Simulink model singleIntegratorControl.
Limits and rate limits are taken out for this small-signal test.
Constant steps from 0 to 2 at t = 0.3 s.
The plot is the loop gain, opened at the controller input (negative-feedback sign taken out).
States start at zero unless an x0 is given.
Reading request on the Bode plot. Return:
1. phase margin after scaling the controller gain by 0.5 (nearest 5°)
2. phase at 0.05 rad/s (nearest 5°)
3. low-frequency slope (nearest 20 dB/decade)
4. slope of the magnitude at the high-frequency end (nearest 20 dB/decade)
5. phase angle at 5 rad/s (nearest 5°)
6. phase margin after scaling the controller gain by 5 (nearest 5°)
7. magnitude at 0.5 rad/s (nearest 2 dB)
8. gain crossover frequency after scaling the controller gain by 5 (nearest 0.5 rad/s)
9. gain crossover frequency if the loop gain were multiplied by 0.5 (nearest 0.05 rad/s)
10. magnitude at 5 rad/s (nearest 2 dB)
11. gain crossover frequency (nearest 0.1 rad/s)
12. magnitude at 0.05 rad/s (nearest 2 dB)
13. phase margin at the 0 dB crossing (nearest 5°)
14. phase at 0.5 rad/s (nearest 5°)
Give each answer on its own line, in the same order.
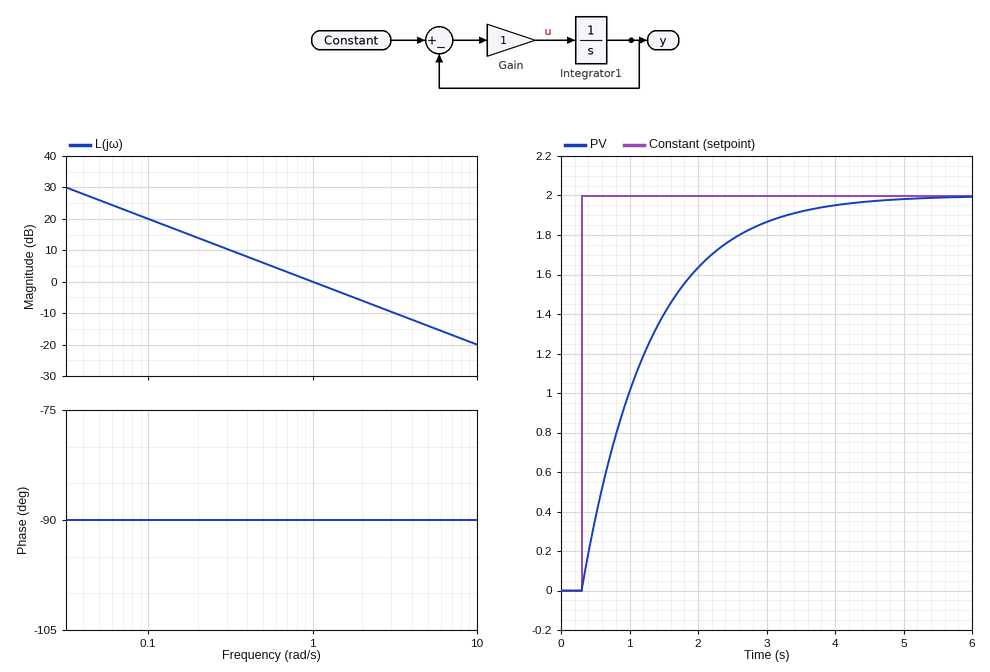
90°
-90°
-20 dB/decade
-20 dB/decade
-90°
90°
6 dB
5.0 rad/s
0.50 rad/s
-14 dB
1.0 rad/s
26 dB
90°
-90°
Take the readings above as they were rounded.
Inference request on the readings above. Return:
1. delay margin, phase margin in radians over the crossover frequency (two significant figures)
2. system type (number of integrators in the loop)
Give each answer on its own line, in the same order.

1.6 s
1
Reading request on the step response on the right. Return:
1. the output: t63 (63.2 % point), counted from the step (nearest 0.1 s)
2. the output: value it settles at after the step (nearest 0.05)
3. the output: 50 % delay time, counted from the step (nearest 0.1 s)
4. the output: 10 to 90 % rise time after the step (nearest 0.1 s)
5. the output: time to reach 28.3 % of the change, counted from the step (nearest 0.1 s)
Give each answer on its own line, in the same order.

1.0 s
2.00
0.7 s
2.2 s
0.3 s
